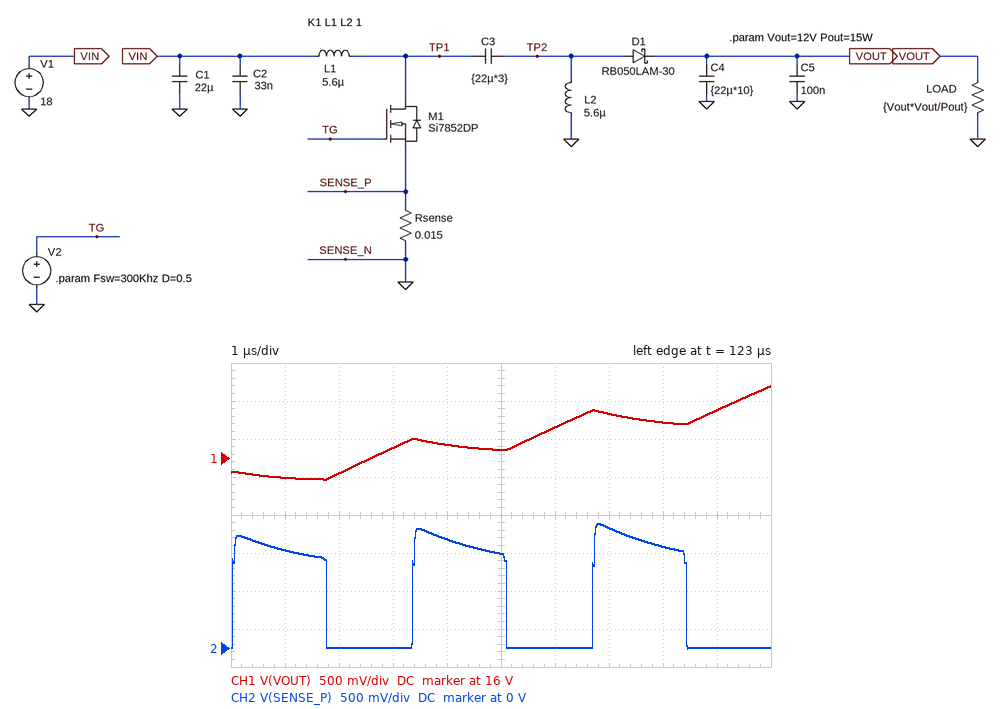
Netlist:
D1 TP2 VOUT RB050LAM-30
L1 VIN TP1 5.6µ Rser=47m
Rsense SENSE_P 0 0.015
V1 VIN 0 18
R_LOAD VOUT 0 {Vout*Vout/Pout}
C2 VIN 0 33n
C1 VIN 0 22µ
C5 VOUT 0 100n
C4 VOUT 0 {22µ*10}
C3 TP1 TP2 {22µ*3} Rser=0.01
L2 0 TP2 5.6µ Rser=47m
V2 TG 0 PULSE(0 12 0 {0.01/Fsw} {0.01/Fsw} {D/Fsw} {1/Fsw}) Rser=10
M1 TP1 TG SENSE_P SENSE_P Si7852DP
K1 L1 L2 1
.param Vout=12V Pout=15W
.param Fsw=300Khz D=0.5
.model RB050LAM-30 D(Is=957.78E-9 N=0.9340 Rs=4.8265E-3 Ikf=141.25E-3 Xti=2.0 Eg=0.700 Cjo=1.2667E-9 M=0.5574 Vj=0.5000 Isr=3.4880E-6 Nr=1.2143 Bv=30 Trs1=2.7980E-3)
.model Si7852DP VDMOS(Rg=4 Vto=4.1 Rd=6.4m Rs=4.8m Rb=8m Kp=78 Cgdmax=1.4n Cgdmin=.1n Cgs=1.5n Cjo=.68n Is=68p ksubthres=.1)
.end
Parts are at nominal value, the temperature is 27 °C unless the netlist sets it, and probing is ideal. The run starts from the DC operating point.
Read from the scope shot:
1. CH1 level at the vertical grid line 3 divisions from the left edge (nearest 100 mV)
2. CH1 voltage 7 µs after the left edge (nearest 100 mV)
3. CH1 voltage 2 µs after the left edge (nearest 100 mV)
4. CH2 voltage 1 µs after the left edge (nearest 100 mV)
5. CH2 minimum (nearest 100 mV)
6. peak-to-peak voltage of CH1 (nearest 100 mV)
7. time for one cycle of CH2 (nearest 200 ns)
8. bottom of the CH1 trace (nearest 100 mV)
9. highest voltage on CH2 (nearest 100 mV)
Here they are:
16.1 V
16.6 V
15.8 V
1.3 V
0 V
1.2 V
3.4 µs
15.7 V
1.6 V
